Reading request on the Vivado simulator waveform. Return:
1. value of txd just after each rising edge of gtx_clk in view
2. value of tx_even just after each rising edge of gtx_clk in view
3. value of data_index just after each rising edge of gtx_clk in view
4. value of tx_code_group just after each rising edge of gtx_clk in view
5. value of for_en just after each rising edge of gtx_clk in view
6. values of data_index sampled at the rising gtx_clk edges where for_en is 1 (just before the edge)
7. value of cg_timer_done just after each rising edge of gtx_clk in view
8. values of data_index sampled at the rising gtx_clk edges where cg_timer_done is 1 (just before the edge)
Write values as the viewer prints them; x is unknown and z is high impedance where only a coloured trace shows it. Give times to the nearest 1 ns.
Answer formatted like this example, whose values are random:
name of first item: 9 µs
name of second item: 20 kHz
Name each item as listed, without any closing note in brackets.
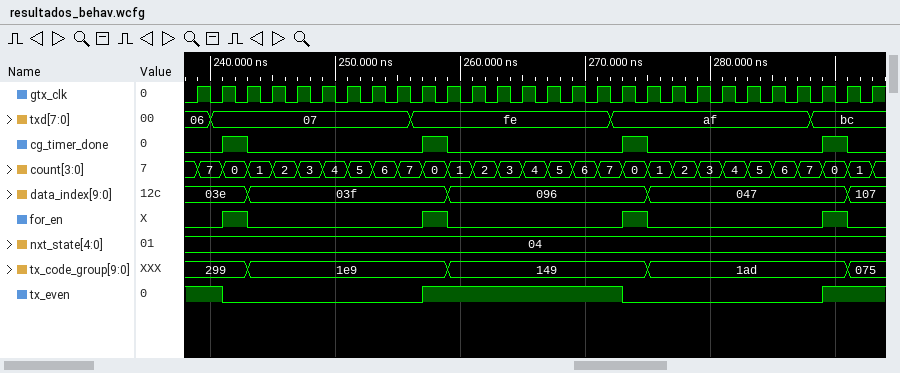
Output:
value of txd just after each rising edge of gtx_clk in view: 06, 07, 07, 07, 07, 07, 07, 07, 07, fe, fe, fe, fe, fe, fe, fe, fe, af, af, af, af, af, af, af, af, bc, bc, bc
value of tx_even just after each rising edge of gtx_clk in view: 1 0 0 0 0 0 0 0 0 1 1 1 1 1 1 1 1 0 0 0 0 0 0 0 0 1 1 1
value of data_index just after each rising edge of gtx_clk in view: 03e, 03e, 03f, 03f, 03f, 03f, 03f, 03f, 03f, 03f, 096, 096, 096, 096, 096, 096, 096, 096, 047, 047, 047, 047, 047, 047, 047, 047, 107, 107
value of tx_code_group just after each rising edge of gtx_clk in view: 299, 299, 1e9, 1e9, 1e9, 1e9, 1e9, 1e9, 1e9, 1e9, 149, 149, 149, 149, 149, 149, 149, 149, 1ad, 1ad, 1ad, 1ad, 1ad, 1ad, 1ad, 1ad, 075, 075
value of for_en just after each rising edge of gtx_clk in view: 0 1 0 0 0 0 0 0 0 1 0 0 0 0 0 0 0 1 0 0 0 0 0 0 0 1 0 0
values of data_index sampled at the rising gtx_clk edges where for_en is 1: 03e, 03f, 096, 047
value of cg_timer_done just after each rising edge of gtx_clk in view: 0 1 0 0 0 0 0 0 0 1 0 0 0 0 0 0 0 1 0 0 0 0 0 0 0 1 0 0
values of data_index sampled at the rising gtx_clk edges where cg_timer_done is 1: 03e, 03f, 096, 047
